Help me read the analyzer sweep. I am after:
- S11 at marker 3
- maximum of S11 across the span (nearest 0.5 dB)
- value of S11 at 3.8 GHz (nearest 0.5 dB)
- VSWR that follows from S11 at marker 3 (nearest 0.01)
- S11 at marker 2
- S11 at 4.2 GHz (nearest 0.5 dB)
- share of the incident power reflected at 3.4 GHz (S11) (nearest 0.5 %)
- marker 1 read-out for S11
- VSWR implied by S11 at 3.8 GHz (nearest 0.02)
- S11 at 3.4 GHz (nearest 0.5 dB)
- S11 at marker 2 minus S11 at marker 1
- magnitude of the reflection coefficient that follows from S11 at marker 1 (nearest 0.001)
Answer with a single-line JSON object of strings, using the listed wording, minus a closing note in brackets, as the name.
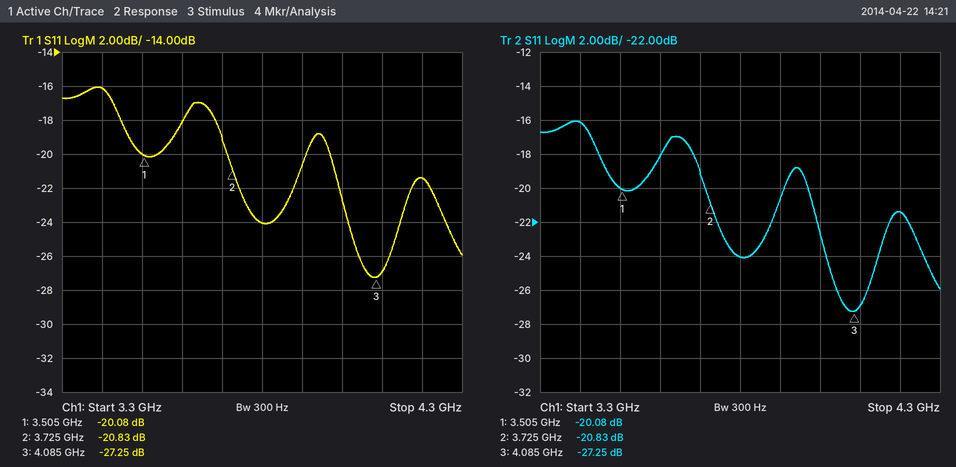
{"S11 at marker 3": "-27.25 dB", "maximum of S11 across the span": "-16.0 dB", "value of S11 at 3.8 GHz": "-24.0 dB", "VSWR that follows from S11 at marker 3": "1.09", "S11 at marker 2": "-20.83 dB", "S11 at 4.2 GHz": "-21.5 dB", "share of the incident power reflected at 3.4 GHz (S11)": "2.5 %", "marker 1 read-out for S11": "-20.08 dB", "VSWR implied by S11 at 3.8 GHz": "1.14", "S11 at 3.4 GHz": "-16.0 dB", "S11 at marker 2 minus S11 at marker 1": "-0.75 dB", "magnitude of the reflection coefficient that follows from S11 at marker 1": "0.099"}
